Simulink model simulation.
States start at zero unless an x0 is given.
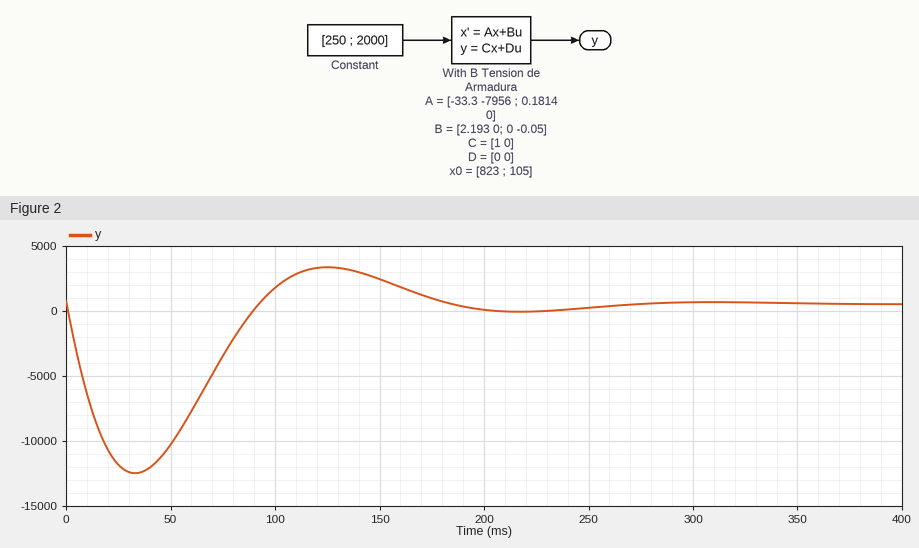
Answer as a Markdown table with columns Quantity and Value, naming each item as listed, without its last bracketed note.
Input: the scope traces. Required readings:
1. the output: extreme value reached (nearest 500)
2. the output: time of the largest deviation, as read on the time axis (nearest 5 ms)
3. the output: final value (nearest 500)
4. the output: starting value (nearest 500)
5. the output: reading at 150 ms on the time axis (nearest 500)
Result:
| Quantity | Value |
|---|---|
| the output: extreme value reached | -12500 |
| the output: time of the largest deviation, as read on the time axis | 35 ms |
| the output: final value | 500 |
| the output: starting value | 1000 |
| the output: reading at 150 ms on the time axis | 2500 |
